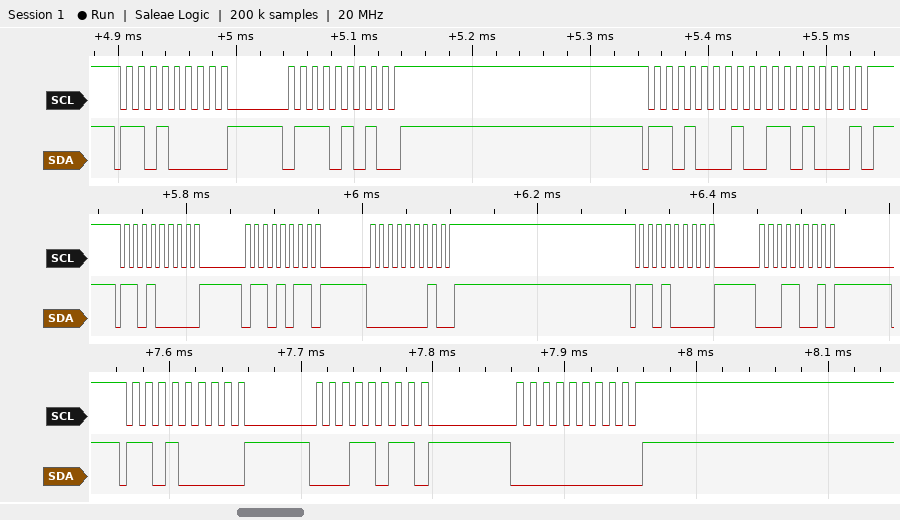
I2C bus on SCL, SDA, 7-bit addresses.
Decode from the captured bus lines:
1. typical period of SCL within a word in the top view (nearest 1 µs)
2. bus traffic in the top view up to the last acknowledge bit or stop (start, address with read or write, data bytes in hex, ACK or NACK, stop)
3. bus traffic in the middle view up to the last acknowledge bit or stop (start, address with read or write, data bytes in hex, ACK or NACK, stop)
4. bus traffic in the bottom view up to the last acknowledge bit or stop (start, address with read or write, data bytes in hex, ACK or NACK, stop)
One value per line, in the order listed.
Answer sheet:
10 µs
start, address 68 write ACK, 75 ACK, stop, start, address 68 read ACK, 68 NACK, stop
start, address 68 write ACK, 6B ACK, 01 ACK, stop, start, address 68 write ACK, 19 ACK
start, address 68 write ACK, 1B ACK, 00 ACK, stop
